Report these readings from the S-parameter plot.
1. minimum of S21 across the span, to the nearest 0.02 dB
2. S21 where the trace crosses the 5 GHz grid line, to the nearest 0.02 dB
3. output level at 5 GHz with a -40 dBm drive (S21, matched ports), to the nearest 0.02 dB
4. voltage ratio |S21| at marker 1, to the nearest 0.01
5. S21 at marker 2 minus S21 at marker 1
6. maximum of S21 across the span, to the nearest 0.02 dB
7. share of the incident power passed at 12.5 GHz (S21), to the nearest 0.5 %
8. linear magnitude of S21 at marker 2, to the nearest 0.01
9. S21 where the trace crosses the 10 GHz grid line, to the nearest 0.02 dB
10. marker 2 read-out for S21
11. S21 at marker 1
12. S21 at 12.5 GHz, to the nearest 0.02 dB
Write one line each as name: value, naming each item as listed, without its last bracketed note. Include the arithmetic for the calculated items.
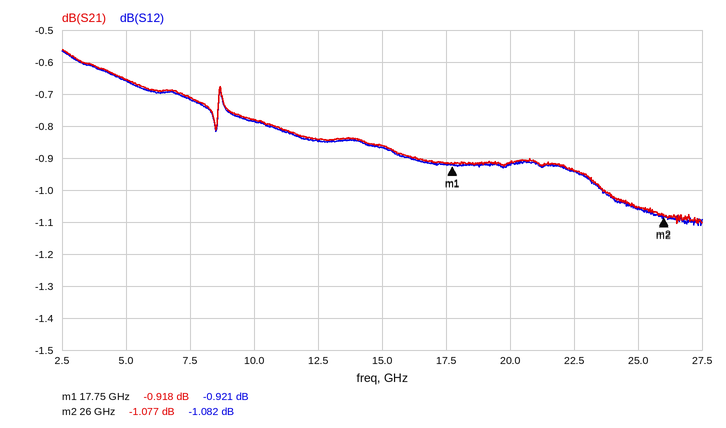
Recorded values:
minimum of S21 across the span, to the nearest 0.02 dB: -1.10 dB
S21 where the trace crosses the 5 GHz grid line, to the nearest 0.02 dB: -0.66 dB
output level at 5 GHz with a -40 dBm drive (S21, matched ports), to the nearest 0.02 dB: -40 dBm + (-0.66 dB) = -40.66 dBm
voltage ratio |S21| at marker 1, to the nearest 0.01: 10^(-0.918/20) ≈ 0.90
S21 at marker 2 minus S21 at marker 1: -1.077 − (-0.918) = -0.159 dB
maximum of S21 across the span, to the nearest 0.02 dB: -0.56 dB
share of the incident power passed at 12.5 GHz (S21), to the nearest 0.5 %: 10^(-0.84/10) ≈ 82.4 %, so 82.5 % to the nearest 0.5 %
linear magnitude of S21 at marker 2, to the nearest 0.01: 10^(-1.077/20) ≈ 0.88
S21 where the trace crosses the 10 GHz grid line, to the nearest 0.02 dB: -0.78 dB
marker 2 read-out for S21: -1.077 dB
S21 at marker 1: -0.918 dB
S21 at 12.5 GHz, to the nearest 0.02 dB: -0.84 dB
